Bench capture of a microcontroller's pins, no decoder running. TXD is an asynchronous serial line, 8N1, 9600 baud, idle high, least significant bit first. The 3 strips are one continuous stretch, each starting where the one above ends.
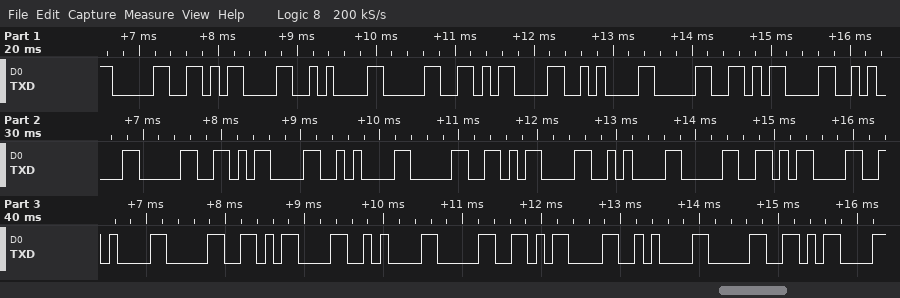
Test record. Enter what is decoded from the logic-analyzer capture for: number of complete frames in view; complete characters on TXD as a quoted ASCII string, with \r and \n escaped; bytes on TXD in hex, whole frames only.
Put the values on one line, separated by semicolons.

26; "0\r\n0\r\n0\r\n0\r\n0\r\n0\r\n0\r\n0\r\n0\r"; 0x30 0x0D 0x0A 0x30 0x0D 0x0A 0x30 0x0D 0x0A 0x30 0x0D 0x0A 0x30 0x0D 0x0A 0x30 0x0D 0x0A 0x30 0x0D 0x0A 0x30 0x0D 0x0A 0x30 0x0D
